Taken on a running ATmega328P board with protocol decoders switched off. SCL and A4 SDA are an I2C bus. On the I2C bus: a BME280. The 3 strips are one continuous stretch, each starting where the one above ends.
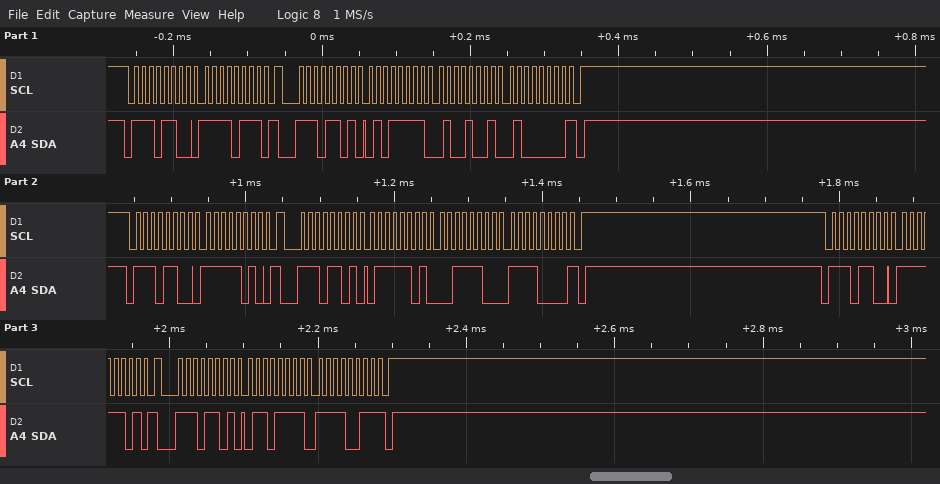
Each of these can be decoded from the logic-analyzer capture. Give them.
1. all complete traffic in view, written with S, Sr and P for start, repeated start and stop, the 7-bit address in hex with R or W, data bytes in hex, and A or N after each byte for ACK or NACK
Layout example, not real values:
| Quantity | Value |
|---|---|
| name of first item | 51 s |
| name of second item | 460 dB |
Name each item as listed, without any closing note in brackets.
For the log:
| Quantity | Value |
|---|---|
| all complete traffic in view, written with S, Sr and P for start, repeated start and stop, the 7-bit address in hex with R or W, data bytes in hex, and A or N after each byte for ACK or NACK | S 76W A F7 A Sr 76R A 5F A 49 A 40 N P S 76W A FA A Sr 76R A 7D A 3C A F0 N P S 76W A FD A Sr 76R A 6F A F3 N P |
